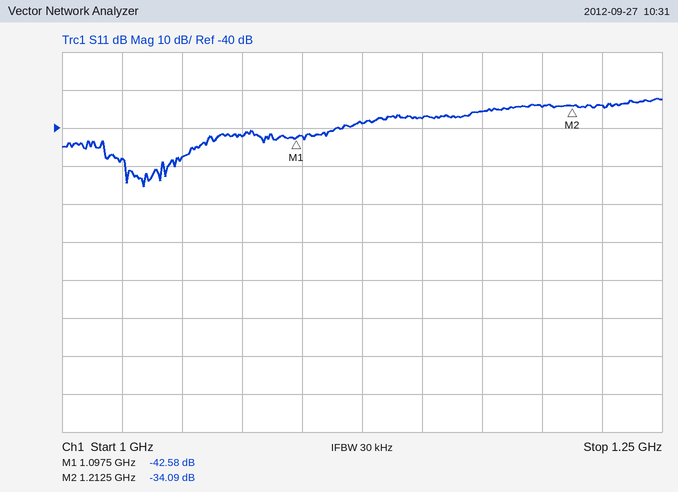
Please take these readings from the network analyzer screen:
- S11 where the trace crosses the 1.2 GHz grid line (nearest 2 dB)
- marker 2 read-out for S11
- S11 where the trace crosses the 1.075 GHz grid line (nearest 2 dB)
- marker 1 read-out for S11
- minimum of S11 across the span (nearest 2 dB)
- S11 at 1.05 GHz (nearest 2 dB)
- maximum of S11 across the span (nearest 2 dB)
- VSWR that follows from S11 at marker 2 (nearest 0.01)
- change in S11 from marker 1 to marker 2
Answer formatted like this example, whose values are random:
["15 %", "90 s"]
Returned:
["-34 dB", "-34.09 dB", "-42 dB", "-42.58 dB", "-56 dB", "-48 dB", "-32 dB", "1.04", "8.49 dB"]
